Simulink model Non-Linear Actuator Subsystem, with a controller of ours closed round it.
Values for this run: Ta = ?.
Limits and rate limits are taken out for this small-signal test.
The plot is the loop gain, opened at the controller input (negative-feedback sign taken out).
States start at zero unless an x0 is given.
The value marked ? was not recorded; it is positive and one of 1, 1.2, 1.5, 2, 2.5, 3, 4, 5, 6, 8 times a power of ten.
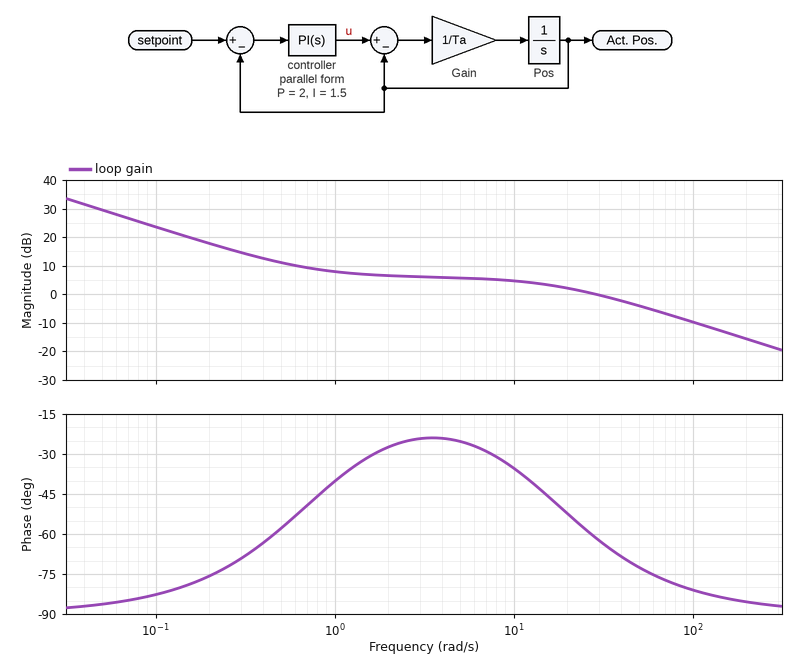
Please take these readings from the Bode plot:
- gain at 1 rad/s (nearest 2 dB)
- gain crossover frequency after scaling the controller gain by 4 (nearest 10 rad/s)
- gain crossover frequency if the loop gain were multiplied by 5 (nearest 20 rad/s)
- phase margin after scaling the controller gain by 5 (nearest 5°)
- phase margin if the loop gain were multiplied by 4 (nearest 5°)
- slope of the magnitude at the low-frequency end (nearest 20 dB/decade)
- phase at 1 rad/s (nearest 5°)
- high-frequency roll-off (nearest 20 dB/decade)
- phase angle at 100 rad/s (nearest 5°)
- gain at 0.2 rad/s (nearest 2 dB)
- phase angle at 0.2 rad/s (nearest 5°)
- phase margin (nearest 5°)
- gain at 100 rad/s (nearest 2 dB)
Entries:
8 dB
130 rad/s
160 rad/s
95°
95°
-20 dB/decade
-40°
-20 dB/decade
-80°
18 dB
-75°
120°
-10 dB
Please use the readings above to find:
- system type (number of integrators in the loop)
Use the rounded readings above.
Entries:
1
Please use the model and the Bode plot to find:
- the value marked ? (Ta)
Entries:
0.06
